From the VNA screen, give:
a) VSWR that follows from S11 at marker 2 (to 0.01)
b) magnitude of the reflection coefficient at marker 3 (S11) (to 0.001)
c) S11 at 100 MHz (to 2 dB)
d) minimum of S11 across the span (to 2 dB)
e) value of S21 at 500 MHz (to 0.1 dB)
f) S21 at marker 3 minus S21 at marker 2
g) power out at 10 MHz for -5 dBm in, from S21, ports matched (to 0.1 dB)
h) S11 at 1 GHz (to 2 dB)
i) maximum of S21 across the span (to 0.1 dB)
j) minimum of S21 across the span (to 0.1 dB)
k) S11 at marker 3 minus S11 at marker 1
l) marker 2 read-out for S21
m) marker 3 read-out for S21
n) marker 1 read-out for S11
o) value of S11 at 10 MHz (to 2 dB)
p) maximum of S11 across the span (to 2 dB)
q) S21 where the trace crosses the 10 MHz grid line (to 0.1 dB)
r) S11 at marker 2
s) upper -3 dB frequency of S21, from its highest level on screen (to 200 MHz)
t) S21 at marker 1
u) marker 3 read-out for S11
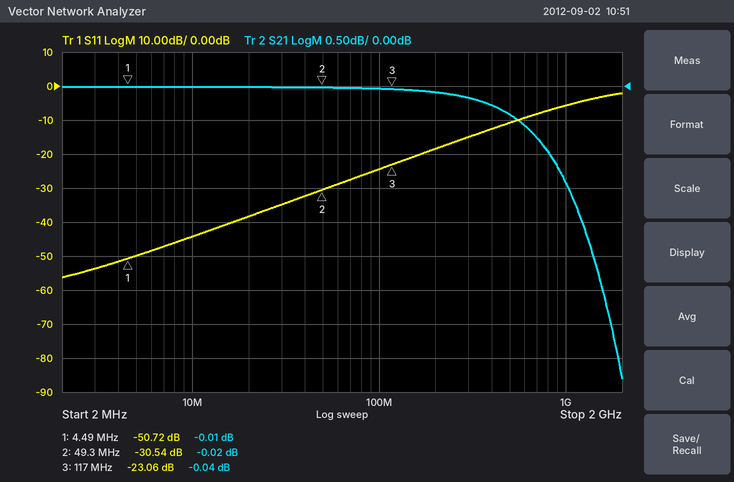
1.06
0.070
-24 dB
-56 dB
-0.4 dB
-0.02 dB
-5.0 dBm
-6 dB
0.0 dB
-4.3 dB
27.66 dB
-0.02 dB
-0.04 dB
-50.72 dB
-44 dB
-2 dB
0.0 dB
-30.54 dB
1.6 GHz
-0.01 dB
-23.06 dB
